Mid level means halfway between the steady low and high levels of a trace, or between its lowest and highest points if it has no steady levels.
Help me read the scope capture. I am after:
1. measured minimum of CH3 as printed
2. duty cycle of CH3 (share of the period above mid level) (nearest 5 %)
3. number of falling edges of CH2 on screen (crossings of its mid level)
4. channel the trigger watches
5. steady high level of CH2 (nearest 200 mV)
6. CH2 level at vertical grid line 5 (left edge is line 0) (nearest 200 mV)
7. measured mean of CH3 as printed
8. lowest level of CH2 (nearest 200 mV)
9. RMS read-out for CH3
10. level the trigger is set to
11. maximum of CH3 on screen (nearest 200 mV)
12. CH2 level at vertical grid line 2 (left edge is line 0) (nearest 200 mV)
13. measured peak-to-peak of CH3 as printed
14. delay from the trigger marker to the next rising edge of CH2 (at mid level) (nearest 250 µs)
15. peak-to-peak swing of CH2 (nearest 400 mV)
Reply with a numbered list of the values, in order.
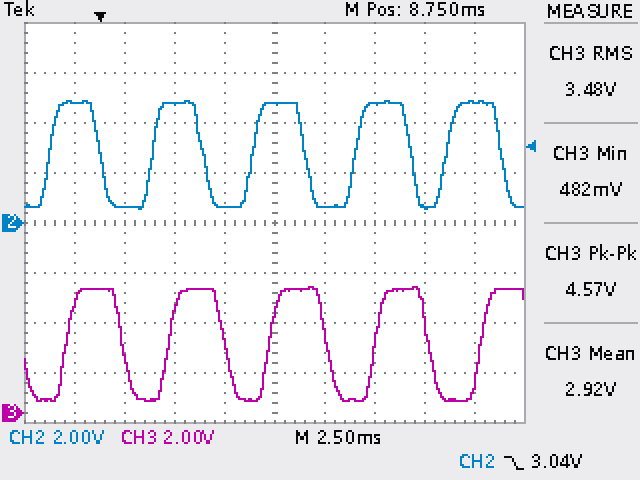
1. 482 mV
2. 55 %
3. 5
4. CH2
5. 4.8 V
6. 4.8 V
7. 2.92 V
8. 600 mV
9. 3.48 V
10. 3.04 V
11. 5.0 V
12. 600 mV
13. 4.57 V
14. 2.75 ms
15. 4.4 V
